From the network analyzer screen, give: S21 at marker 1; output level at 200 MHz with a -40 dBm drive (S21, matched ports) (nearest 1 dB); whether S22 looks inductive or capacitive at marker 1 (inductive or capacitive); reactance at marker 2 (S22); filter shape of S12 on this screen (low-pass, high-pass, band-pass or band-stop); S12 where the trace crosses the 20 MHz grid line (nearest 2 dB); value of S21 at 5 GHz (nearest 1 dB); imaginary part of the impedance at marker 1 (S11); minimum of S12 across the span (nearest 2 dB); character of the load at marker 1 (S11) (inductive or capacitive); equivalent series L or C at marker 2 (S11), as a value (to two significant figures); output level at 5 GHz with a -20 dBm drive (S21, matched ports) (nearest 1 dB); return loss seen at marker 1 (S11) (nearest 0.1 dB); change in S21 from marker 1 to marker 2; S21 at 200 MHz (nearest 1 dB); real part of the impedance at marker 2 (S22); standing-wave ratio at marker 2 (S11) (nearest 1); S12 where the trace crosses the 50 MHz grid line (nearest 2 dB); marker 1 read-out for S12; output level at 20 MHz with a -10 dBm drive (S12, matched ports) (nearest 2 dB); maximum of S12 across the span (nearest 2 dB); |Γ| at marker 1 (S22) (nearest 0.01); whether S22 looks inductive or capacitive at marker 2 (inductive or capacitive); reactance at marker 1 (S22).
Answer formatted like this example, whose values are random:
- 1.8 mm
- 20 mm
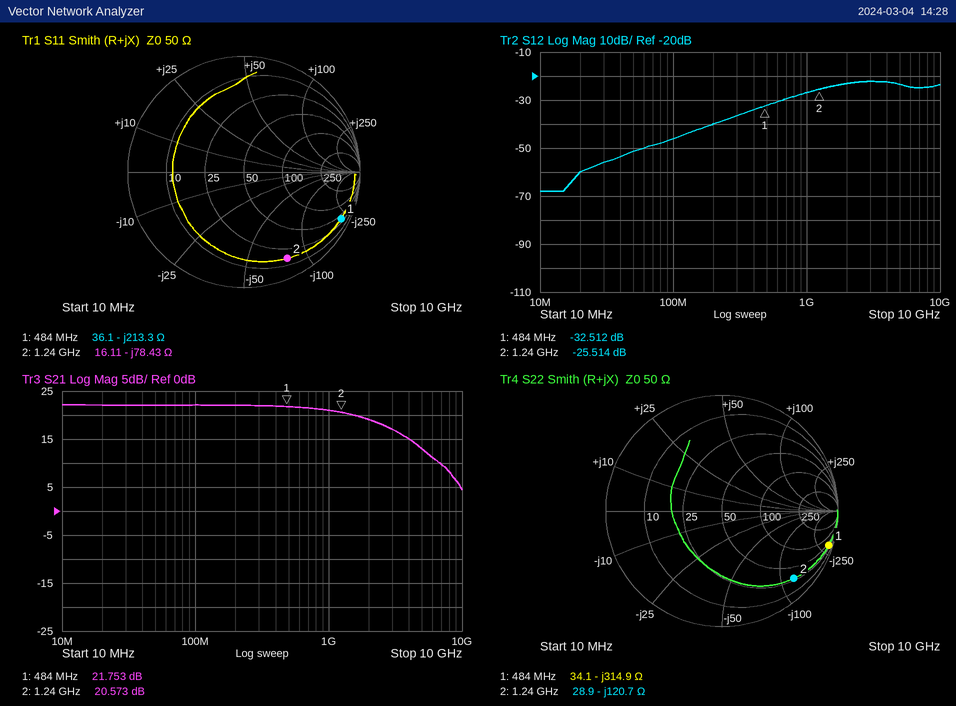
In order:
- 21.753 dB
- -18 dBm
- capacitive
- -120.7 Ω
- high-pass
- -60 dB
- 13 dB
- -213.3 Ω
- -68 dB
- capacitive
- 1.6 pF
- -7 dBm
- 0.6 dB
- -1.180 dB
- 22 dB
- 28.9 Ω
- 11
- -52 dB
- -32.512 dB
- -70 dBm
- -22 dB
- 0.97
- capacitive
- -314.9 Ω
